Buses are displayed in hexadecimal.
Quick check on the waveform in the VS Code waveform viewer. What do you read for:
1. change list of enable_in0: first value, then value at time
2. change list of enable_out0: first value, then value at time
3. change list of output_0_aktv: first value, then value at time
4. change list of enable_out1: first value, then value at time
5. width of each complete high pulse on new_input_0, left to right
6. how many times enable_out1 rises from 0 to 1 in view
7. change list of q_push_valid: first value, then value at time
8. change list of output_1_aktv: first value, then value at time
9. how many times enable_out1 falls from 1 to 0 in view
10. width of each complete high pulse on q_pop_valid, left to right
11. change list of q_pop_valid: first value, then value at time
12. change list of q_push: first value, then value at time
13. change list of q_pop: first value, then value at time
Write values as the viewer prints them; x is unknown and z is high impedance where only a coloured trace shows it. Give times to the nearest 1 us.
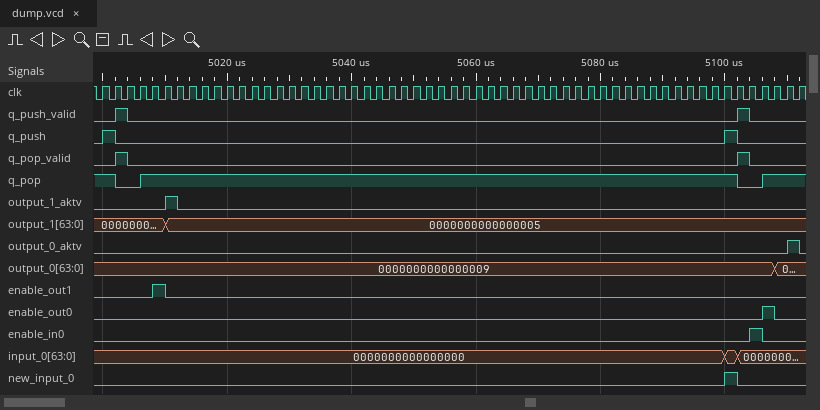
0, 1 at 5104 us, 0 at 5106 us
0, 1 at 5106 us, 0 at 5108 us
0, 1 at 5110 us, 0 at 5112 us
0, 1 at 5008 us, 0 at 5010 us
2 us
1
0, 1 at 5002 us, 0 at 5004 us, 1 at 5102 us, 0 at 5104 us
0, 1 at 5010 us, 0 at 5012 us
1
2 us, 2 us
0, 1 at 5002 us, 0 at 5004 us, 1 at 5102 us, 0 at 5104 us
0, 1 at 5000 us, 0 at 5002 us, 1 at 5100 us, 0 at 5102 us
1, 0 at 5002 us, 1 at 5006 us, 0 at 5102 us, 1 at 5106 us
